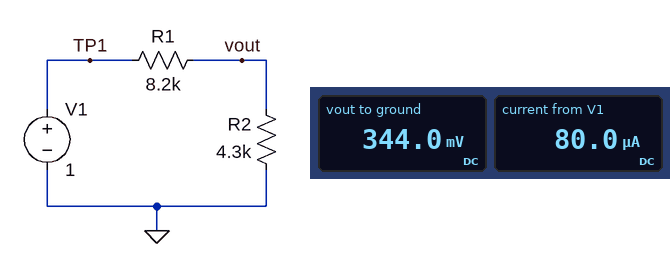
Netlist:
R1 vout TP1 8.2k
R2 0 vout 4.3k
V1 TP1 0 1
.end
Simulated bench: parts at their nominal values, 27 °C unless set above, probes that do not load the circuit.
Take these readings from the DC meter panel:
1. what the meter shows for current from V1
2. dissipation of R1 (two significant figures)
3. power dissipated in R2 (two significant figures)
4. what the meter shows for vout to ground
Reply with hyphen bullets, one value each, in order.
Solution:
- 80.0 µA
- 52 µW
- 28 µW
- 344.0 mV
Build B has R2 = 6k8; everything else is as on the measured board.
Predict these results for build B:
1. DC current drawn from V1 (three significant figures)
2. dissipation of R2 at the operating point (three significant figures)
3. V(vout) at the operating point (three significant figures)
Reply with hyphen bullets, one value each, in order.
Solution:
- 66.7 µA
- 30.2 µW
- 453 mV
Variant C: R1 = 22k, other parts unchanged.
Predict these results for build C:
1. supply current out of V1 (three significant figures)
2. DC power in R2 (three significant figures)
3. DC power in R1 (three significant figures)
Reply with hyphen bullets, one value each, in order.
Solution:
- 38.0 µA
- 6.22 µW
- 31.8 µW
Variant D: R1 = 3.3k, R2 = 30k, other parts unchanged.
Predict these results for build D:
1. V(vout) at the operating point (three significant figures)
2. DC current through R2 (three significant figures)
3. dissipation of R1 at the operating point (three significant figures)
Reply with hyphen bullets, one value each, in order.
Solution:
- 901 mV
- 30.0 µA
- 2.98 µW
